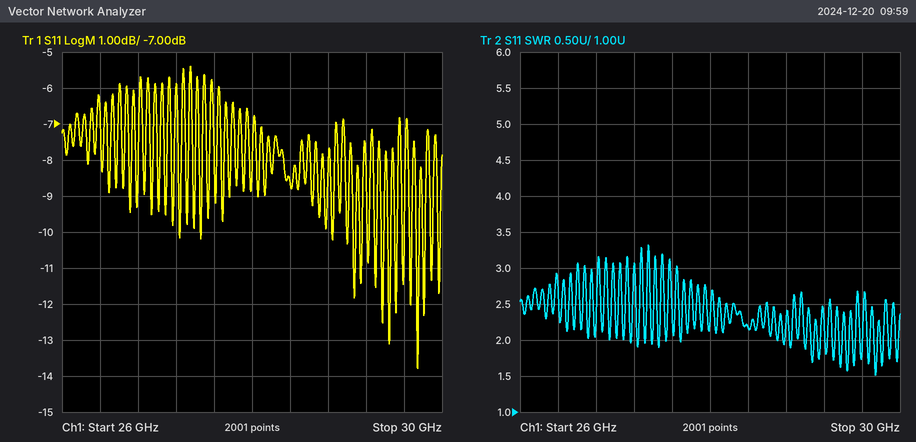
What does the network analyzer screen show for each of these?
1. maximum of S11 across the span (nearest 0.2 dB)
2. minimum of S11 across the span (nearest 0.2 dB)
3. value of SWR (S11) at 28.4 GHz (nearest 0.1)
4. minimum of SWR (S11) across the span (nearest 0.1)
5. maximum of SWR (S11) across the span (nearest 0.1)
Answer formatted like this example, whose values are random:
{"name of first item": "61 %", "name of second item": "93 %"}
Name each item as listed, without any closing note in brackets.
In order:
{"maximum of S11 across the span": "-5.4 dB", "minimum of S11 across the span": "-13.8 dB", "value of SWR (S11) at 28.4 GHz": "2.2", "minimum of SWR (S11) across the span": "1.5", "maximum of SWR (S11) across the span": "3.3"}
